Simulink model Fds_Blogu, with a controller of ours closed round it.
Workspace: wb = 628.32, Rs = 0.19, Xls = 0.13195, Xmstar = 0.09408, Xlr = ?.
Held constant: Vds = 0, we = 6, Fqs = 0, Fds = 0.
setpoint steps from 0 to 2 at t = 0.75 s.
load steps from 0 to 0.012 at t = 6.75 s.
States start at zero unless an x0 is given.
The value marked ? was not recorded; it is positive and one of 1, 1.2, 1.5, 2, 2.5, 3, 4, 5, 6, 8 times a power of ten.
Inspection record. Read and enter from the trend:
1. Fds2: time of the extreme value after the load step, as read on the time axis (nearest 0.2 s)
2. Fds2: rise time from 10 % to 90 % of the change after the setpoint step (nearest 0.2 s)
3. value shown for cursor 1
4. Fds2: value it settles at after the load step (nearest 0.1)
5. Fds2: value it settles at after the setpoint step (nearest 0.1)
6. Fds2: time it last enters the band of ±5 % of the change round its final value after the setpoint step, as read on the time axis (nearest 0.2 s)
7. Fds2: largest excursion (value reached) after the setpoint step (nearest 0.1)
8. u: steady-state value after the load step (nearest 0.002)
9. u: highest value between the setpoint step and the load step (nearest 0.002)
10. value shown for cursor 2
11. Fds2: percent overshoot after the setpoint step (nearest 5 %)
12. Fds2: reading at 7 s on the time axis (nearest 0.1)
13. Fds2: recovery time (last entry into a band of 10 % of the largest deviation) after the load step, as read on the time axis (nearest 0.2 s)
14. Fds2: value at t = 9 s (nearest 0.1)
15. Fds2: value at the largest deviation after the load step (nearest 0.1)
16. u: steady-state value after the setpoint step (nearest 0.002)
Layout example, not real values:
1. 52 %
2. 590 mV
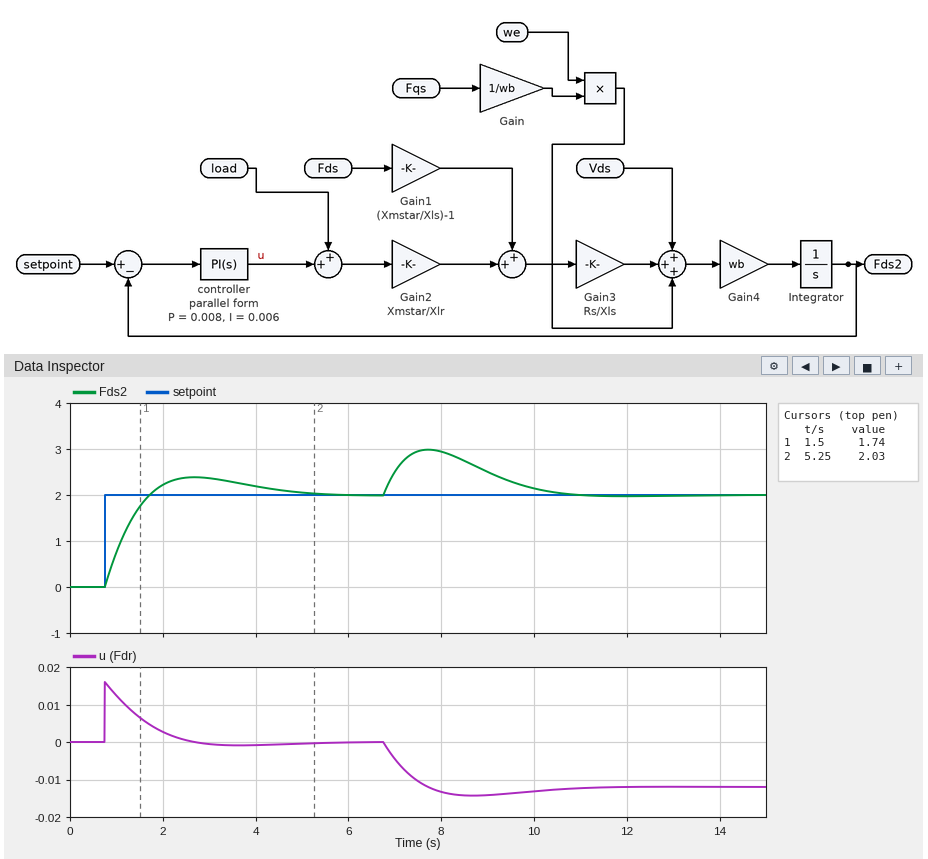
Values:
1. 7.8 s
2. 0.8 s
3. 1.74
4. 2.0
5. 2.0
6. 4.6 s
7. 2.4
8. -0.012
9. 0.016
10. 2.03
11. 20 %
12. 2.5
13. 10.2 s
14. 2.5
15. 3.0
16. 0.000
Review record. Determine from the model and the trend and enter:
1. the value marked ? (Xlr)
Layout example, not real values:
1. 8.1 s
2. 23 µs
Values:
1. 0.4
